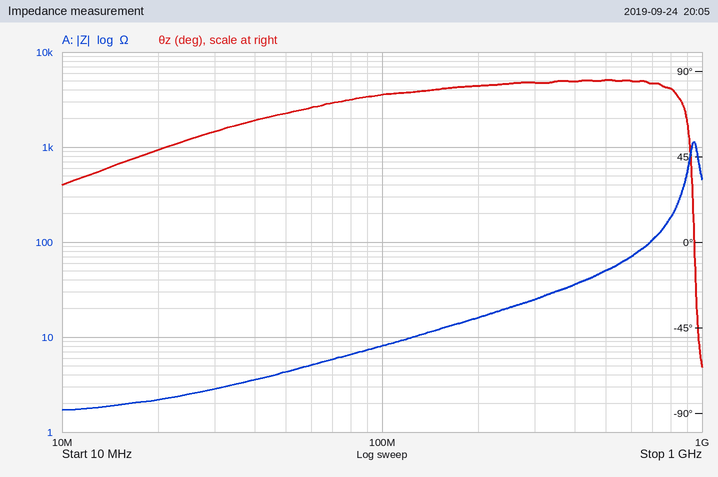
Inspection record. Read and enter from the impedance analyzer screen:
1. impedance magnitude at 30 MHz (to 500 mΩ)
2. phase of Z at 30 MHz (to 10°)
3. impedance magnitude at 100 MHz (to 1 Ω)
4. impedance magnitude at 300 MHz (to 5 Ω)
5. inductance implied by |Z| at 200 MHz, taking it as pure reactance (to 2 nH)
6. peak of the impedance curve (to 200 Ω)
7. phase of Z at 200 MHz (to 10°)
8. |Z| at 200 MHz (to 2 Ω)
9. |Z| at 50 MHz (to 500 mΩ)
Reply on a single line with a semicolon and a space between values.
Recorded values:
3.0 Ω; 60°; 8 Ω; 25 Ω; 12 nH; 1.2 kΩ; 80°; 16 Ω; 4.5 Ω
